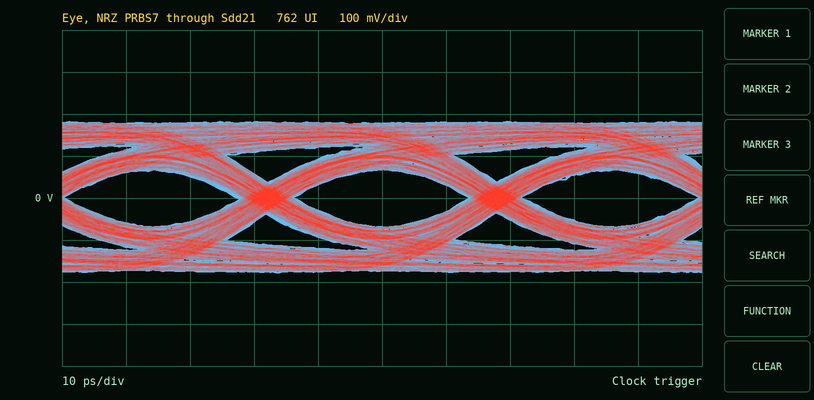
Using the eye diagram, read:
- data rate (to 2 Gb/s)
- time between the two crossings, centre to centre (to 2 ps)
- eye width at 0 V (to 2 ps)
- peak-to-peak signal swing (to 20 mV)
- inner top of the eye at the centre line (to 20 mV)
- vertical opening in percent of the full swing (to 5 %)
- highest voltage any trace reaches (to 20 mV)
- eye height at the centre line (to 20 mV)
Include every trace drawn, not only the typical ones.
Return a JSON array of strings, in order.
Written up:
["28 Gb/s", "36 ps", "28 ps", "360 mV", "60 mV", "40 %", "180 mV", "140 mV"]
